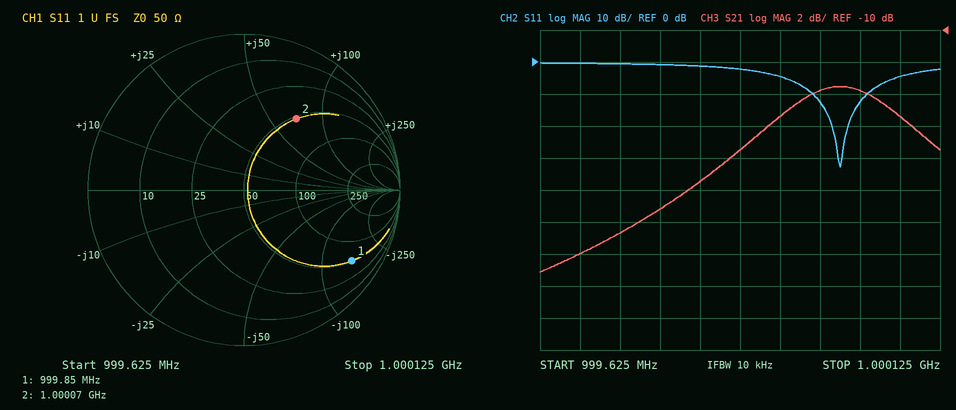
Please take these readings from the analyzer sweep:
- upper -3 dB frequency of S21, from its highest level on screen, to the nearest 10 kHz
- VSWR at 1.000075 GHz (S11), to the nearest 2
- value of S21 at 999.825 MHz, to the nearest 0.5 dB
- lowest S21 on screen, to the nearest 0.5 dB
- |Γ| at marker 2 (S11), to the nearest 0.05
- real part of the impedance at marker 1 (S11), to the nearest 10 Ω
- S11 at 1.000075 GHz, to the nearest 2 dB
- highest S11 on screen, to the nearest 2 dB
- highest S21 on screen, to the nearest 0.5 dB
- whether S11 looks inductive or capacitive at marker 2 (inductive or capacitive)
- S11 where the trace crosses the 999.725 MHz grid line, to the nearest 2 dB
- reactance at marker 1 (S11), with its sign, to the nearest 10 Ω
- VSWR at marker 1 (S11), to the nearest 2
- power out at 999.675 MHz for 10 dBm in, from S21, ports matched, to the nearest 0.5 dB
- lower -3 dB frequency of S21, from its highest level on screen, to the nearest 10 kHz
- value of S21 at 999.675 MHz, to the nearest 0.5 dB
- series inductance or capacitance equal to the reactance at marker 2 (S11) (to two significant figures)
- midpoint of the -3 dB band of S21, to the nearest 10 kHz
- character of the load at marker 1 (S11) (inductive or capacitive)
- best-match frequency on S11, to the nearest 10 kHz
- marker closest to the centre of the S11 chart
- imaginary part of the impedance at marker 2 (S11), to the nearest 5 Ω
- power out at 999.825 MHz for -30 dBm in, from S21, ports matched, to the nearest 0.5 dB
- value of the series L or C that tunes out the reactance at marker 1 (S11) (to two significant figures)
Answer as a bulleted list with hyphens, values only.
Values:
- 1.00010 GHz
- 4
- -19.5 dB
- -25.0 dB
- 0.55
- 50 Ω
- -4 dB
- 0 dB
- -13.5 dB
- inductive
- 0 dB
- -150 Ω
- 10
- -14.0 dBm
- 999.90 MHz
- -24.0 dB
- 11 nH
- 1.00000 GHz
- capacitive
- 1.00000 GHz
- marker 2
- +70 Ω
- -49.5 dBm
- 24 nH
